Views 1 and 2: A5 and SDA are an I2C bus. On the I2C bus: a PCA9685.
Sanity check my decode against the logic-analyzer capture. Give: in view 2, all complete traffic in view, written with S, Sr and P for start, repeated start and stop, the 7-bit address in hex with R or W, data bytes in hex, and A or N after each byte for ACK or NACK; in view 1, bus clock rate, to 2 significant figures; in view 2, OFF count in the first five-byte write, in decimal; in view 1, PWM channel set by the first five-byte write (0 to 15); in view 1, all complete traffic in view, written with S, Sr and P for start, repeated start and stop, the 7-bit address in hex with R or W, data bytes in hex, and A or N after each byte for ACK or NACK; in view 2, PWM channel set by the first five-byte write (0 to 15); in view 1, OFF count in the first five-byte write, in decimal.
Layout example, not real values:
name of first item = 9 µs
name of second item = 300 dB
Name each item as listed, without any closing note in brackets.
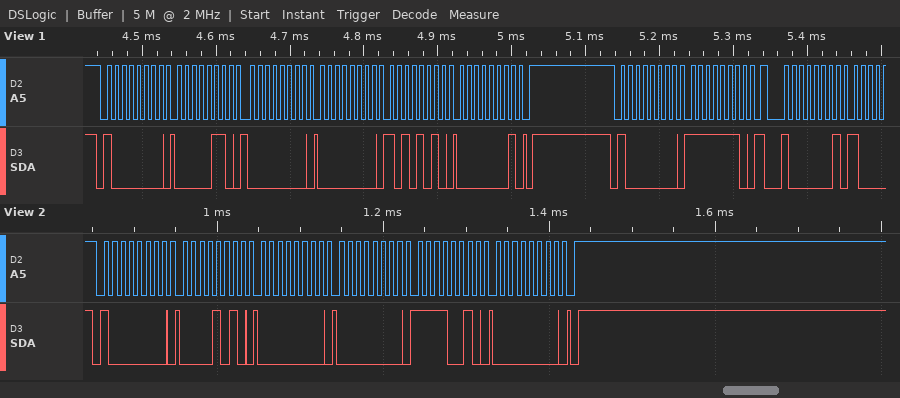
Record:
in view 2, all complete traffic in view, written with S, Sr and P for start, repeated start and stop, the 7-bit address in hex with R or W, data bytes in hex, and A or N after each byte for ACK or NACK = S 40W A 0A A 00 A 00 A F2 A 00 A P
in view 1, bus clock rate, to 2 significant figures = 100 kHz
in view 2, OFF count in the first five-byte write, in decimal = 242
in view 1, PWM channel set by the first five-byte write = 0
in view 1, all complete traffic in view, written with S, Sr and P for start, repeated start and stop, the 7-bit address in hex with R or W, data bytes in hex, and A or N after each byte for ACK or NACK = S 40W A 06 A 00 A 00 A AA A 01 A P S 40W A FE A Sr 40R A
in view 2, PWM channel set by the first five-byte write = 1
in view 1, OFF count in the first five-byte write, in decimal = 426
